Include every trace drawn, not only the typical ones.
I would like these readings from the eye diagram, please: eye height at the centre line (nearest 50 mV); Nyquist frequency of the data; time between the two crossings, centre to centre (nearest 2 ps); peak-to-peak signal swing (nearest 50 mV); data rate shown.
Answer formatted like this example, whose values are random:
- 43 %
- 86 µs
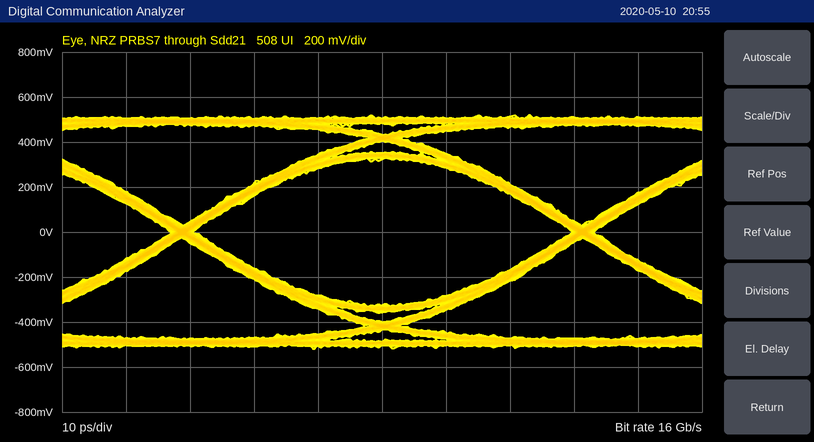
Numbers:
- 650 mV
- 8 GHz
- 62 ps
- 1.05 V
- 16 Gb/s
